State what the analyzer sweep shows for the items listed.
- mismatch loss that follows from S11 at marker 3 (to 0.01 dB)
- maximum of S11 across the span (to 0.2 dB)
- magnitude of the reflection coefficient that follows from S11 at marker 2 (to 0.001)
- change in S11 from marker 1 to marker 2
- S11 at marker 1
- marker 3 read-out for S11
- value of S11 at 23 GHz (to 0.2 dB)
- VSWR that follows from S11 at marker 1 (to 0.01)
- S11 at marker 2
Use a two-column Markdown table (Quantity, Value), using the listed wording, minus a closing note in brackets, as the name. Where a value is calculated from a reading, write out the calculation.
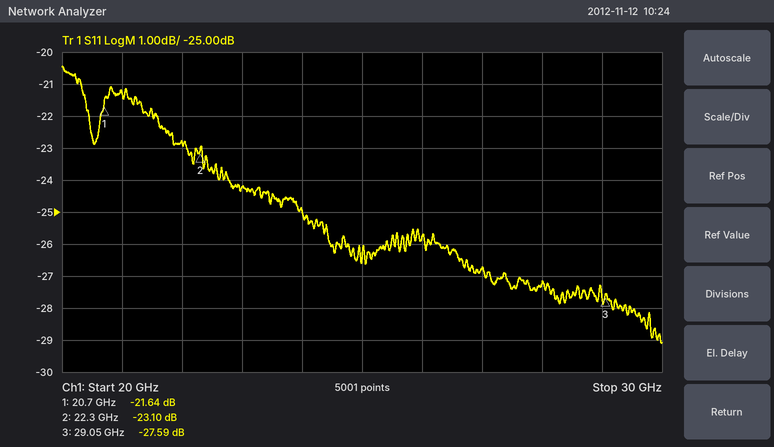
| Quantity | Value |
|---|---|
| mismatch loss that follows from S11 at marker 3 | −10 log10(1 − 10^(-27.59/10)) ≈ 0.01 dB |
| maximum of S11 across the span | -20.4 dB |
| magnitude of the reflection coefficient that follows from S11 at marker 2 | 10^(-23.1/20) ≈ 0.070 |
| change in S11 from marker 1 to marker 2 | -23.1 − (-21.64) = -1.46 dB |
| S11 at marker 1 | -21.64 dB |
| marker 3 read-out for S11 | -27.59 dB |
| value of S11 at 23 GHz | -24.2 dB |
| VSWR that follows from S11 at marker 1 | (1 + 0.0828)/(1 − 0.0828) ≈ 1.18 |
| S11 at marker 2 | -23.10 dB |
